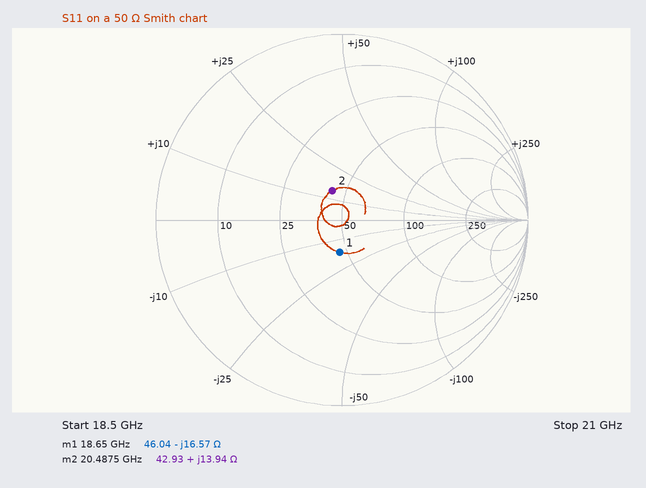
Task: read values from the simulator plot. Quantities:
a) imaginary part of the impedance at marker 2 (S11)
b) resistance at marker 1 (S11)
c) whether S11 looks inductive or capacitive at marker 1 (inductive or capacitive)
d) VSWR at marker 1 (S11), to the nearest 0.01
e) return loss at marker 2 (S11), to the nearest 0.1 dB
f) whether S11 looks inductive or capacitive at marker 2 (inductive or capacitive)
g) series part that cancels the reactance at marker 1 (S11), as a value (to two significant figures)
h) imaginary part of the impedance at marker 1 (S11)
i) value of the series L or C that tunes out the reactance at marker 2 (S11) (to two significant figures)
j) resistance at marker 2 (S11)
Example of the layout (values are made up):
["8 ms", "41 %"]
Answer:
["+13.94 Ω", "46.04 Ω", "capacitive", "1.42", "15.6 dB", "inductive", "140 pH", "-16.57 Ω", "560 fF", "42.93 Ω"]
